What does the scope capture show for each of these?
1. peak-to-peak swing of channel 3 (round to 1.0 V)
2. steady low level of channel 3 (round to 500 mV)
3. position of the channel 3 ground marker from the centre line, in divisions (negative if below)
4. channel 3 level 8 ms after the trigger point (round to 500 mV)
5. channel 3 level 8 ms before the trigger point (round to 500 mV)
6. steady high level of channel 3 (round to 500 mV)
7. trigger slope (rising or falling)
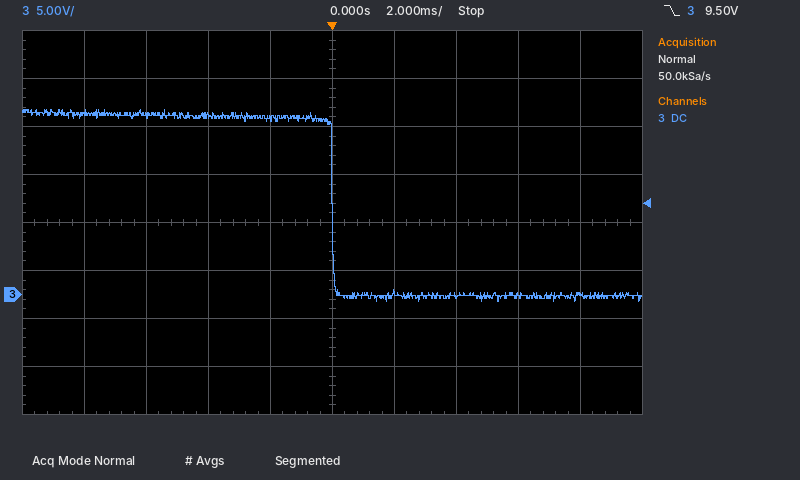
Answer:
20.0 V
0.0 V
-1.5 div
0.0 V
19.0 V
18.5 V
falling
